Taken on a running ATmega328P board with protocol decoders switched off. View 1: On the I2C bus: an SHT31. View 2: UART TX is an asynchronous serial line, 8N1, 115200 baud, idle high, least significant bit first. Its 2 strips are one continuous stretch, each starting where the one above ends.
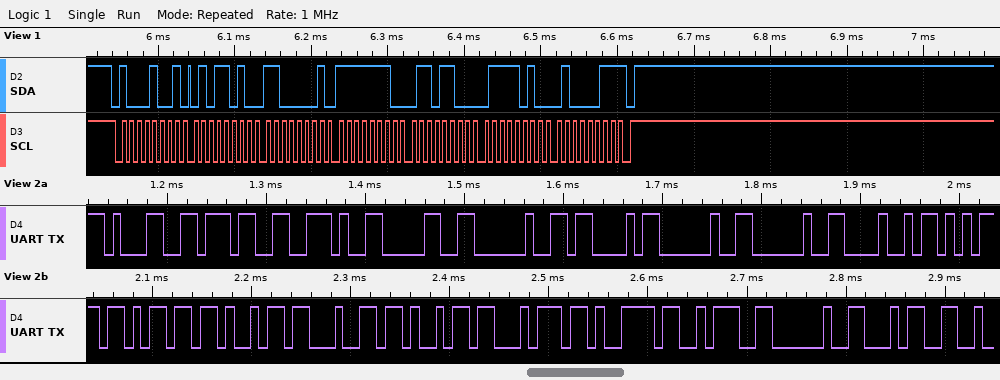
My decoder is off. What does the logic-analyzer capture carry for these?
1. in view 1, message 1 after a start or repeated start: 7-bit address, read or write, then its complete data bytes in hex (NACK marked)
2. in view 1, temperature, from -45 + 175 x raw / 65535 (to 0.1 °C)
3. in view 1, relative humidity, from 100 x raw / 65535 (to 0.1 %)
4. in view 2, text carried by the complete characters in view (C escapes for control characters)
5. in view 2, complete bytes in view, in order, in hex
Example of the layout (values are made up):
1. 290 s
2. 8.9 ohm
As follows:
1. 0x44 read: 5A C1 FE 6C 7A 43 NACK
2. 17.0 °C
3. 42.4 %
4. "17.0 C  Humidity: 4"
5. 31 37 2E 30 20 43 20 20 48 75 6D 69 64 69 74 79 3A 20 34
